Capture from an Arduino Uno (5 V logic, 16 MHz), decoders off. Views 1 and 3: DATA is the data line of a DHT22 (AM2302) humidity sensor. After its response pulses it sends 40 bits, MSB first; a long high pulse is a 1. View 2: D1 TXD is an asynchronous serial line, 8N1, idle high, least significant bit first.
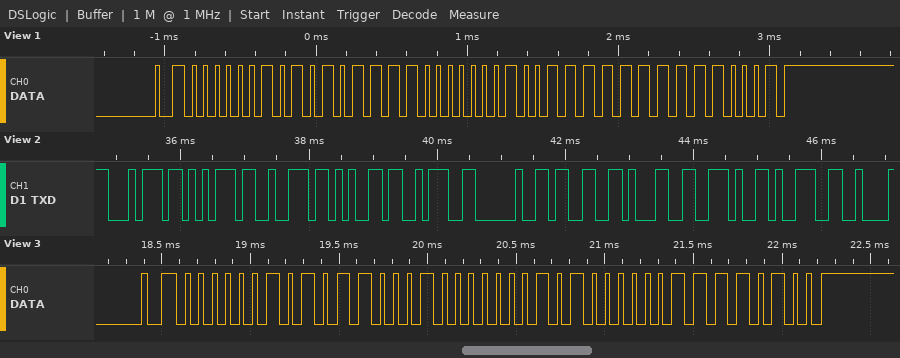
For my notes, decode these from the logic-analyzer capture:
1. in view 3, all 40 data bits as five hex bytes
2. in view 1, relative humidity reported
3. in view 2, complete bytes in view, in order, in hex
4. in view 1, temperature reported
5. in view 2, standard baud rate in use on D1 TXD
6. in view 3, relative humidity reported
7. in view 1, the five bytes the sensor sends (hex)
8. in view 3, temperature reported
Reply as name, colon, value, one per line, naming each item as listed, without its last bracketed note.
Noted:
in view 3, all 40 data bits as five hex bytes: 02 B1 01 40 F4
in view 1, relative humidity reported: 68.7 %
in view 2, complete bytes in view, in order, in hex: 74 75 72 65 3A 20 33 31 2E 39
in view 1, temperature reported: 31.9 °C
in view 2, standard baud rate in use on D1 TXD: 9600 baud
in view 3, relative humidity reported: 68.9 %
in view 1, the five bytes the sensor sends: 02 AF 01 3F F1
in view 3, temperature reported: 32.0 °C
